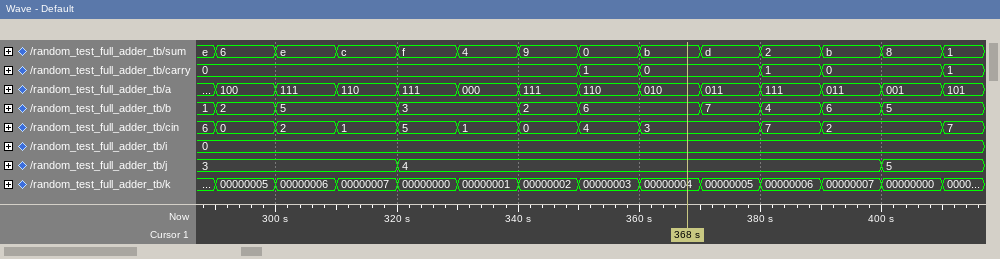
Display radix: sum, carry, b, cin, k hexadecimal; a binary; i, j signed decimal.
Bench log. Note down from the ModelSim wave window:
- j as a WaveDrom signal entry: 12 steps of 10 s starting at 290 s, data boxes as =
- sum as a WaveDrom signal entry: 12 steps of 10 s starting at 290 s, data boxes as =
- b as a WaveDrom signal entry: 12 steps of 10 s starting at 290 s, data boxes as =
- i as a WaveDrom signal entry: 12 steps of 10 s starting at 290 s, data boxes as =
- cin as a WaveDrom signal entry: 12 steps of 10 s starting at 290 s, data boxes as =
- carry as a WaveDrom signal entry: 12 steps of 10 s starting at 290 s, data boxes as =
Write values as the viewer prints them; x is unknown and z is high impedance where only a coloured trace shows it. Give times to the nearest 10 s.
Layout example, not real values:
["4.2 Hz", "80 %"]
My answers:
["{name: 'j', wave: '=..=.......=', data: '3 4 5'}", "{name: 'sum', wave: '============', data: '6 e c f 4 9 0 b d 2 b 8'}", "{name: 'b', wave: '==.=.==.====', data: '2 5 3 2 6 7 4 6 5'}", "{name: 'i', wave: '=...........', data: '0'}", "{name: 'cin', wave: '========.==.', data: '0 2 1 5 1 0 4 3 7 2'}", "{name: 'carry', wave: '=.....==.==.', data: '0 1 0 1 0'}"]
